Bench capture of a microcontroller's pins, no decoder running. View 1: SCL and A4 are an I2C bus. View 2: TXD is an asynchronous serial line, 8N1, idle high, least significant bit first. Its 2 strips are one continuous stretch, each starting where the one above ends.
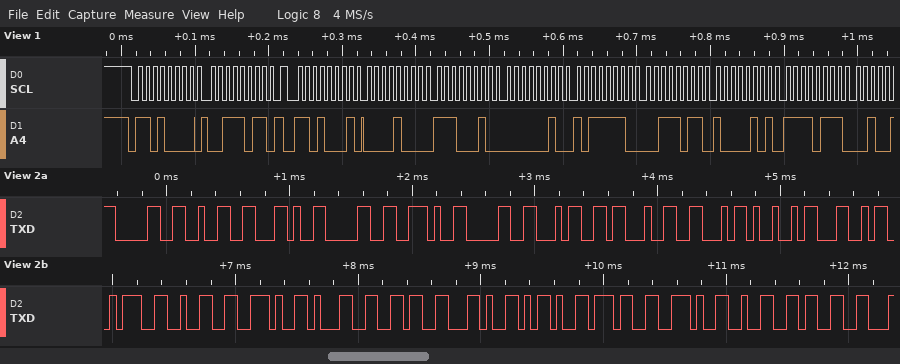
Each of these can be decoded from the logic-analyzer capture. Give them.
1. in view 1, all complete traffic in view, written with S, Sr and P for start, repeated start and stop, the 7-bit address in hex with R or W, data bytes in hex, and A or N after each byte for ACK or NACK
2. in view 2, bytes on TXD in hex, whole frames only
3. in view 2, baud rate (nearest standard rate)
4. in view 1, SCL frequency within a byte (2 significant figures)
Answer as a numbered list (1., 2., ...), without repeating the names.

1. S 68W A 3B A Sr 68R A 08 A E2 A 02 A BE A 3B A 85 A F7 A
2. 30 32 2C 30 2E 30 34 23 46 49 4C 3A 32 2E 31 36 2C 2D 37 2E 32 33
3. 19200 baud
4. 100 kHz
